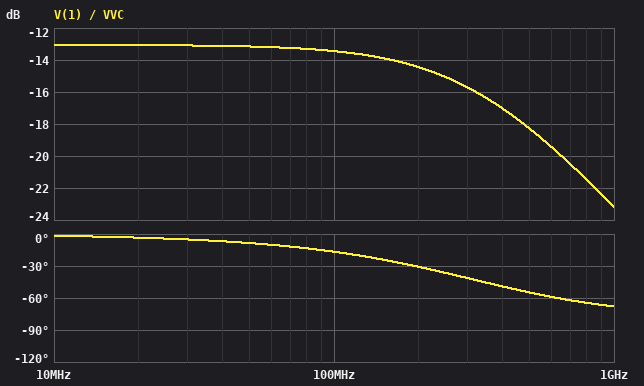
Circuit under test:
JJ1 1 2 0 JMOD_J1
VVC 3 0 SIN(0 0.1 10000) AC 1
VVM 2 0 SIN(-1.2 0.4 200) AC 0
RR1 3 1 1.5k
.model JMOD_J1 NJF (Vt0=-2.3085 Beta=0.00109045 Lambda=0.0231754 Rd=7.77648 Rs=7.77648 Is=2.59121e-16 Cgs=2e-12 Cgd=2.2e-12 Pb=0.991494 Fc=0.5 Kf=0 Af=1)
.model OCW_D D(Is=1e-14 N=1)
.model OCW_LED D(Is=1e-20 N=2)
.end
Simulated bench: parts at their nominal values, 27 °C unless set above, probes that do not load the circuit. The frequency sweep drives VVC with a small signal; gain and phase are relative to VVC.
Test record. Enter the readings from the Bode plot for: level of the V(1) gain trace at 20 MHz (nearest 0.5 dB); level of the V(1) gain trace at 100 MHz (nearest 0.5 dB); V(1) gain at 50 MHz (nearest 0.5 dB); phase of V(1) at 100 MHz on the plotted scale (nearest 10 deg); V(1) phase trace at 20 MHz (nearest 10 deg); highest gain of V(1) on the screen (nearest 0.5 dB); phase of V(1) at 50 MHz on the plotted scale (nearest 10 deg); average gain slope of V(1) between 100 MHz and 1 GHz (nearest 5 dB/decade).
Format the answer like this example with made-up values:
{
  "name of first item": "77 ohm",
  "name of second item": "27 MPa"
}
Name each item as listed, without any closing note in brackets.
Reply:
{
  "level of the V(1) gain trace at 20 MHz": "-13.0 dB",
  "level of the V(1) gain trace at 100 MHz": "-13.5 dB",
  "V(1) gain at 50 MHz": "-13.0 dB",
  "phase of V(1) at 100 MHz on the plotted scale": "-20 deg",
  "V(1) phase trace at 20 MHz": "0 deg",
  "highest gain of V(1) on the screen": "-13.0 dB",
  "phase of V(1) at 50 MHz on the plotted scale": "-10 deg",
  "average gain slope of V(1) between 100 MHz and 1 GHz": "-10 dB/decade"
}
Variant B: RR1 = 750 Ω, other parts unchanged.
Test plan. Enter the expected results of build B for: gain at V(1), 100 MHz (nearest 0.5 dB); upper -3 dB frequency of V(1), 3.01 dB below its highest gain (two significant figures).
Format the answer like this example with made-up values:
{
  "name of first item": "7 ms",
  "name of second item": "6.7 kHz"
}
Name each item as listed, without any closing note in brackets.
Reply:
{
  "gain at V(1), 100 MHz": "-9.0 dB",
  "upper -3 dB frequency of V(1), 3.01 dB below its highest gain": "400 MHz"
}
